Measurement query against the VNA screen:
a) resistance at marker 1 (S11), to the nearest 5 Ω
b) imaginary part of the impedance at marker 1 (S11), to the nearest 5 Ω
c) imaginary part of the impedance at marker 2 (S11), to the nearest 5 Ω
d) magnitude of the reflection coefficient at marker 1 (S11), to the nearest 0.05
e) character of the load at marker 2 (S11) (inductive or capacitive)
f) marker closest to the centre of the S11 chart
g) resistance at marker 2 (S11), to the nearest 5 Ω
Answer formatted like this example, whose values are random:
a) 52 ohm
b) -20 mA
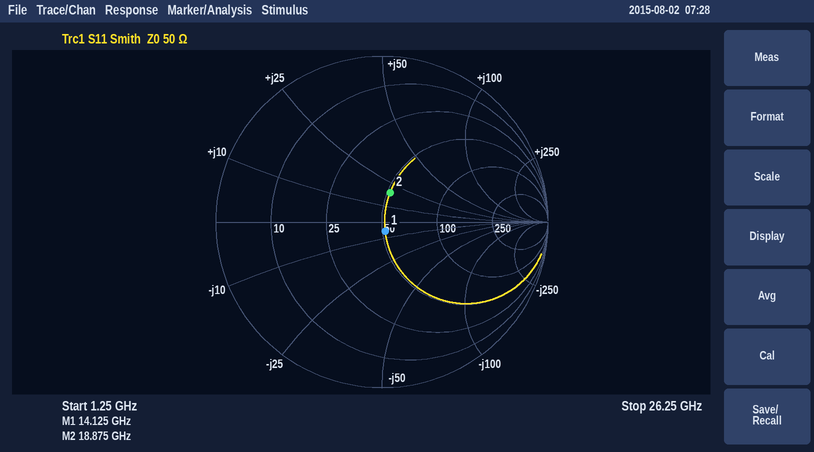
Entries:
a) 50 Ω
b) -5 Ω
c) +20 Ω
d) 0.05
e) inductive
f) marker 1
g) 50 Ω
